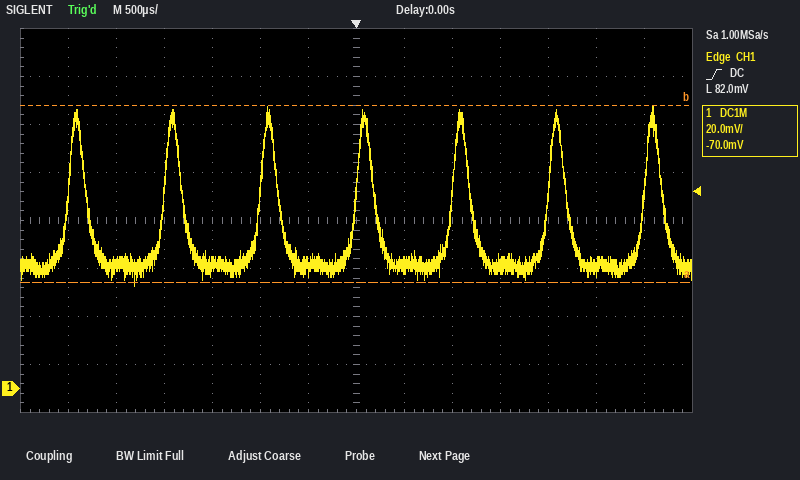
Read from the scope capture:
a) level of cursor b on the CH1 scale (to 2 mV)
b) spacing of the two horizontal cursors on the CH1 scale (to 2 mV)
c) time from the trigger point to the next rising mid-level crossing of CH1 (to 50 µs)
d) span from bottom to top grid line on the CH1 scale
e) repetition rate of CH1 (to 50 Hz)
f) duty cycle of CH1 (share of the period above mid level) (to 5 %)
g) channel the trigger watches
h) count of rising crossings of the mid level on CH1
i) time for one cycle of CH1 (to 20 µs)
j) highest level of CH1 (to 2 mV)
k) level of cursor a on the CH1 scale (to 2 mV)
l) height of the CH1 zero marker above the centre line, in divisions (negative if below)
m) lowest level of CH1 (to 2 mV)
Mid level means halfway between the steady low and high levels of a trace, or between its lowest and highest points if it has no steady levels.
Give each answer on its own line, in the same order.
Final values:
118 mV
74 mV
1.00 ms
160 mV
1.00 kHz
20 %
CH1
7
1.00 ms
118 mV
44 mV
-3.5 div
42 mV
